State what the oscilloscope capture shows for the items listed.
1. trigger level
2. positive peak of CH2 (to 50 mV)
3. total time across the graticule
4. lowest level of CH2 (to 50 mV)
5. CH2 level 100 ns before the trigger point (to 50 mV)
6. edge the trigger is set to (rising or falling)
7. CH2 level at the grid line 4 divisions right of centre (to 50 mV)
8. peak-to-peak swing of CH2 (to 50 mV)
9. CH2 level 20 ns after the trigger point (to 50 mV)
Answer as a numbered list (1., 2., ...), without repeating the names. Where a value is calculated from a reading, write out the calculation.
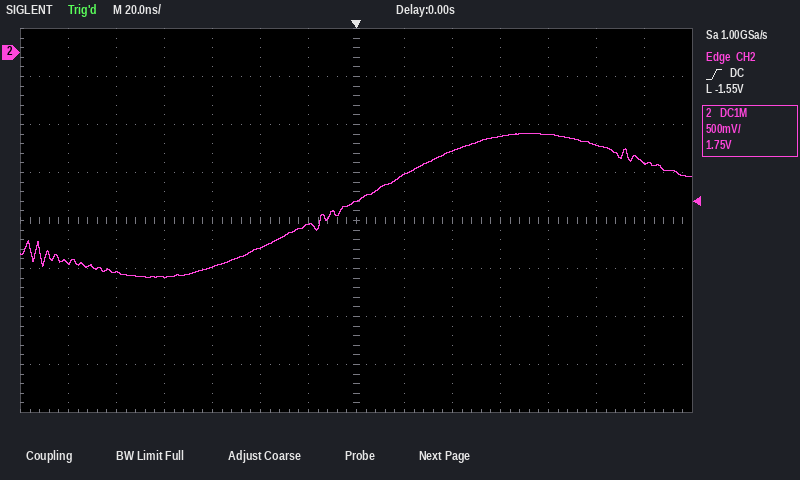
1. -1.55 V
2. -850 mV
3. 280 ns
4. -2.35 V
5. -2.30 V
6. rising
7. -850 mV
8. -850 mV − (-2.35 V) = 1.50 V
9. -1.25 V
